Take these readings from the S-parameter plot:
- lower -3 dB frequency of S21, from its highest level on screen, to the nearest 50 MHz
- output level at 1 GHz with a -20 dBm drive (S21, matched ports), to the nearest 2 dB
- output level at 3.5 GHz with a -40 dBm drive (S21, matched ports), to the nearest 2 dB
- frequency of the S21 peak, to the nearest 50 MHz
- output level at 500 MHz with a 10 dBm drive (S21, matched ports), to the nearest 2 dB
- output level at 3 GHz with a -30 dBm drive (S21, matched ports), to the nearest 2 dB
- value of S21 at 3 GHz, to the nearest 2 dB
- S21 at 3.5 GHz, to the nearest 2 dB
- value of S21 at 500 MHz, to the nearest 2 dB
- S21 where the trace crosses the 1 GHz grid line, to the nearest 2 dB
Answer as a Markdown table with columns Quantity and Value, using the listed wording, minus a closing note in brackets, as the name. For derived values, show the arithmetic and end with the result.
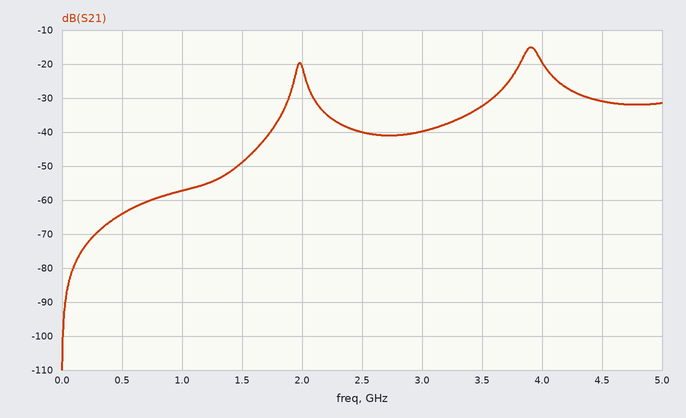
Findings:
| Quantity | Value |
|---|---|
| lower -3 dB frequency of S21, from its highest level on screen, to the nearest 50 MHz | 3.85 GHz |
| output level at 1 GHz with a -20 dBm drive (S21, matched ports), to the nearest 2 dB | -20 dBm + (-58 dB) = -78 dBm |
| output level at 3.5 GHz with a -40 dBm drive (S21, matched ports), to the nearest 2 dB | -40 dBm + (-32 dB) = -72 dBm |
| frequency of the S21 peak, to the nearest 50 MHz | 3.90 GHz |
| output level at 500 MHz with a 10 dBm drive (S21, matched ports), to the nearest 2 dB | 10 dBm + (-64 dB) = -54 dBm |
| output level at 3 GHz with a -30 dBm drive (S21, matched ports), to the nearest 2 dB | -30 dBm + (-40 dB) = -70 dBm |
| value of S21 at 3 GHz, to the nearest 2 dB | -40 dB |
| S21 at 3.5 GHz, to the nearest 2 dB | -32 dB |
| value of S21 at 500 MHz, to the nearest 2 dB | -64 dB |
| S21 where the trace crosses the 1 GHz grid line, to the nearest 2 dB | -58 dB |
